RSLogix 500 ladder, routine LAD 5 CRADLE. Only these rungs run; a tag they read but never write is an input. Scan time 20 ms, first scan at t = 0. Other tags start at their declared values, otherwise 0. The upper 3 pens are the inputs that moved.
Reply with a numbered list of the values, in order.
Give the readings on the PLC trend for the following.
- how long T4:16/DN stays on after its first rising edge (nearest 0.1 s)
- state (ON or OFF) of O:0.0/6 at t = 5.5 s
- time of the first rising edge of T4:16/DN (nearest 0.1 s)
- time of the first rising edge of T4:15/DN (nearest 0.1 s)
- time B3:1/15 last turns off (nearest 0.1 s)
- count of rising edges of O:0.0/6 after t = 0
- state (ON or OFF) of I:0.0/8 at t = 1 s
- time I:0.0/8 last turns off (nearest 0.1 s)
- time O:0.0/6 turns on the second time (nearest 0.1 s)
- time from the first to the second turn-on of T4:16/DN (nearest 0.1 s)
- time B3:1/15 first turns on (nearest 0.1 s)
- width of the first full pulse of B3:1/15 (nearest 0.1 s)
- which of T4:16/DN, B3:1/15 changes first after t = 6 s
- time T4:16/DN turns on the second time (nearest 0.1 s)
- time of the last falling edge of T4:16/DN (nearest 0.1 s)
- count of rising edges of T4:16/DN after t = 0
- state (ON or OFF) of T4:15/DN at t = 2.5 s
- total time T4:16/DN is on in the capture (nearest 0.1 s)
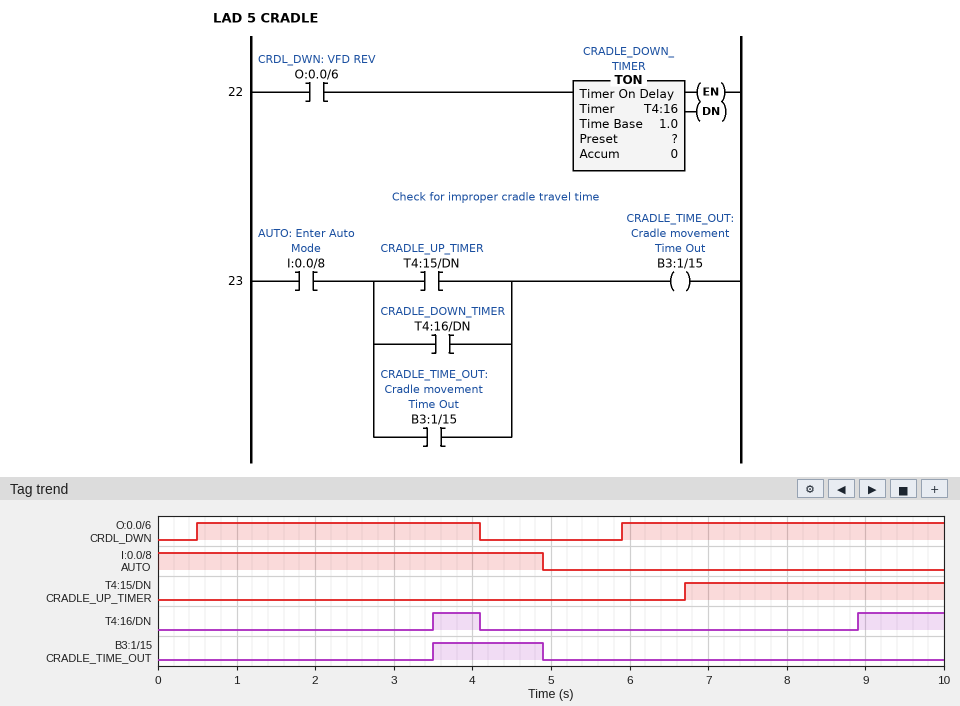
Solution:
1. 0.6 s
2. OFF
3. 3.5 s
4. 6.7 s
5. 4.9 s
6. 2
7. ON
8. 4.9 s
9. 5.9 s
10. 5.4 s
11. 3.5 s
12. 1.4 s
13. T4:16/DN
14. 8.9 s
15. 4.1 s
16. 2
17. OFF
18. 1.7 s
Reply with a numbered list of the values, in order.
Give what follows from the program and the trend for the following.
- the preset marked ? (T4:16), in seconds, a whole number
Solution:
1. 3 s
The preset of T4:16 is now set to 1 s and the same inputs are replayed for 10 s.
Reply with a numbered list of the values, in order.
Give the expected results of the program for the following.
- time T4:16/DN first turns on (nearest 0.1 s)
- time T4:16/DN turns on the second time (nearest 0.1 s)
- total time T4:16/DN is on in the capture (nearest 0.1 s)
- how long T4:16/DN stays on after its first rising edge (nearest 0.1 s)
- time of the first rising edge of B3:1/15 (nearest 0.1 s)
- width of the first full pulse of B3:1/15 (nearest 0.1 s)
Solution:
1. 1.5 s
2. 6.9 s
3. 5.7 s
4. 2.6 s
5. 1.5 s
6. 3.4 s
